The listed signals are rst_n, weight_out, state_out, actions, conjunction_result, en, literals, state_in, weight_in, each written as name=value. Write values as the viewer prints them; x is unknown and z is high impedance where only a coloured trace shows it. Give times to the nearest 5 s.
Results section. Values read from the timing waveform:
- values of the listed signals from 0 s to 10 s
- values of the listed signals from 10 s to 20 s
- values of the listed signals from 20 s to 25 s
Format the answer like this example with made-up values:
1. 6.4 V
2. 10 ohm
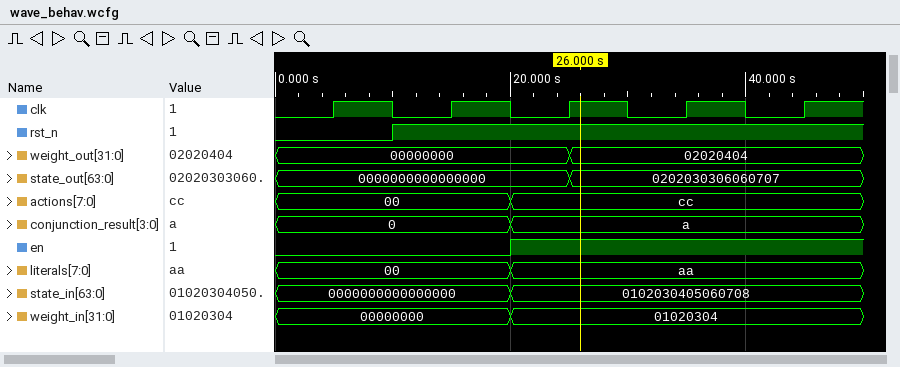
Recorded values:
1. rst_n=0, weight_out=00000000, state_out=0000000000000000, actions=00, conjunction_result=0, en=0, literals=00, state_in=0000000000000000, weight_in=00000000
2. rst_n=1, weight_out=00000000, state_out=0000000000000000, actions=00, conjunction_result=0, en=0, literals=00, state_in=0000000000000000, weight_in=00000000
3. rst_n=1, weight_out=00000000, state_out=0000000000000000, actions=cc, conjunction_result=a, en=1, literals=aa, state_in=0102030405060708, weight_in=01020304
